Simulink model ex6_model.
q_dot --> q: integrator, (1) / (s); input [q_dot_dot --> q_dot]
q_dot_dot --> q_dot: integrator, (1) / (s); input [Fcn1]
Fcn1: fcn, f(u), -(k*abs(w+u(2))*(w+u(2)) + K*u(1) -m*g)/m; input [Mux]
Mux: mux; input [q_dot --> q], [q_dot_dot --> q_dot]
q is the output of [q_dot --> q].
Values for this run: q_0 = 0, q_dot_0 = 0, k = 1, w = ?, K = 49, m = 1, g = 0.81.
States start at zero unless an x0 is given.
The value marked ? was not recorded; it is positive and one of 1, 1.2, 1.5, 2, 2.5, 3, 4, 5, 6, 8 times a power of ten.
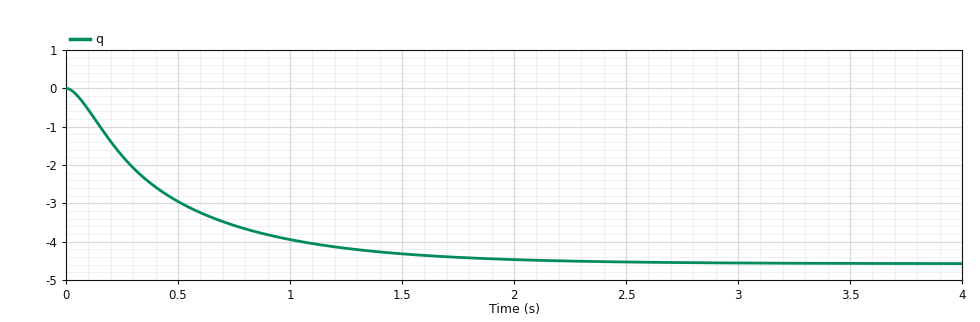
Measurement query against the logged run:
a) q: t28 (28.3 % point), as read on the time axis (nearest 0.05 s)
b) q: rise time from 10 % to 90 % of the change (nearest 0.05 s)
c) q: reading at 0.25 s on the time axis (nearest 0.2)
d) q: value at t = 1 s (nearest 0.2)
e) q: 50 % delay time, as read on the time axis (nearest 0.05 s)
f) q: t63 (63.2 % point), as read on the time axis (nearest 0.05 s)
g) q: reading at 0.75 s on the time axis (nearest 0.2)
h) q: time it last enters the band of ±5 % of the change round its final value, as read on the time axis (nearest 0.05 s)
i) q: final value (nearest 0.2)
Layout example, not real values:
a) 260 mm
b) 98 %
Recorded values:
a) 0.20 s
b) 1.10 s
c) -1.8
d) -4.0
e) 0.35 s
f) 0.50 s
g) -3.6
h) 1.55 s
i) -4.6
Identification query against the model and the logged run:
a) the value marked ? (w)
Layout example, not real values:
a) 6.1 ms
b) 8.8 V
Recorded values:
a) 15
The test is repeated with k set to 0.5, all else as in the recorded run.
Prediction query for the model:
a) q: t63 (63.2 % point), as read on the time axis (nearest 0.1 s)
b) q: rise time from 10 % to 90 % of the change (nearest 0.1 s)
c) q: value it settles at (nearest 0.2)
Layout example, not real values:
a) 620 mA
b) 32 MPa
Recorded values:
a) 0.3 s
b) 0.4 s
c) -2.2
